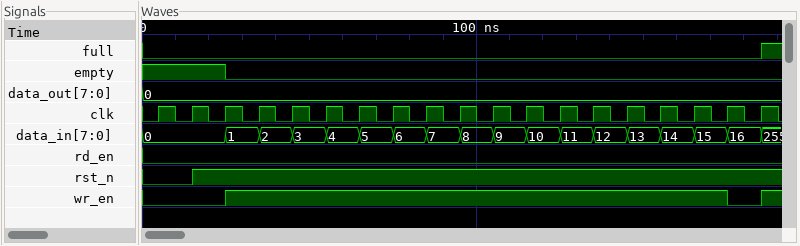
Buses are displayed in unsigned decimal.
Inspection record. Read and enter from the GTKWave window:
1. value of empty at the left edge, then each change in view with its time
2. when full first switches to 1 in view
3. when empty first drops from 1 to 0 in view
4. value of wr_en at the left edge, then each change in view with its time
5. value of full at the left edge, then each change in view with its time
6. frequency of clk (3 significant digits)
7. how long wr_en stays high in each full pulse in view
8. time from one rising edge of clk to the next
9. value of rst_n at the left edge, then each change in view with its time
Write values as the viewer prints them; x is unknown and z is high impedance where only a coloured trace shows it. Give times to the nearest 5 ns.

1, 0 at 25 ns
185 ns
25 ns
0, 1 at 25 ns, 0 at 175 ns, 1 at 185 ns
0, 1 at 185 ns
100 MHz
150 ns
10 ns
0, 1 at 15 ns
